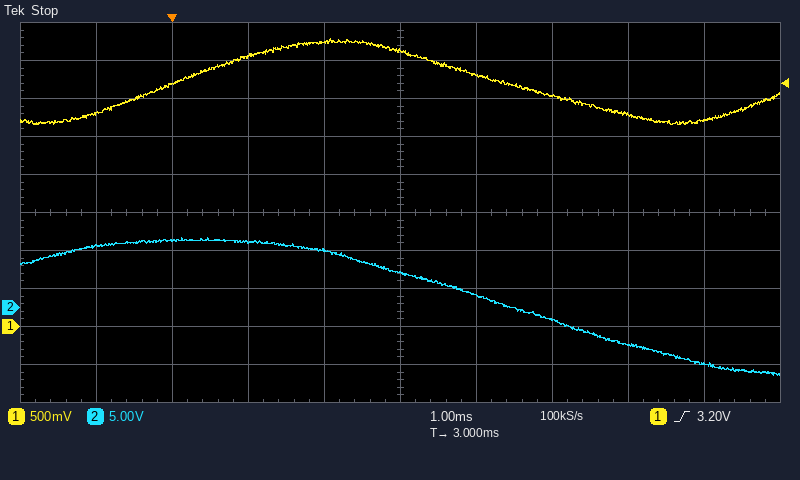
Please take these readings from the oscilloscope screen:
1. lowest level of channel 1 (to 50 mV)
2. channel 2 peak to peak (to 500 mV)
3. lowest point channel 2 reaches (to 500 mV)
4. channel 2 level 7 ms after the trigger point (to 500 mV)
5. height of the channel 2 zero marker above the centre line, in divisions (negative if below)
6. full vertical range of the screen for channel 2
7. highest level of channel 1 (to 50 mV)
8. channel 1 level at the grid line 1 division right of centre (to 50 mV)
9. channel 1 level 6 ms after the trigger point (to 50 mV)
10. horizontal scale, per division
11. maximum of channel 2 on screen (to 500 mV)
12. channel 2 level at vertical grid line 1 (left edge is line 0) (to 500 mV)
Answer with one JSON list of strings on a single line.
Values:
["2.65 V", "18.0 V", "-9.0 V", "-7.5 V", "-2.5 div", "50 V", "3.80 V", "3.30 V", "2.80 V", "1 ms", "9.0 V", "8.0 V"]
